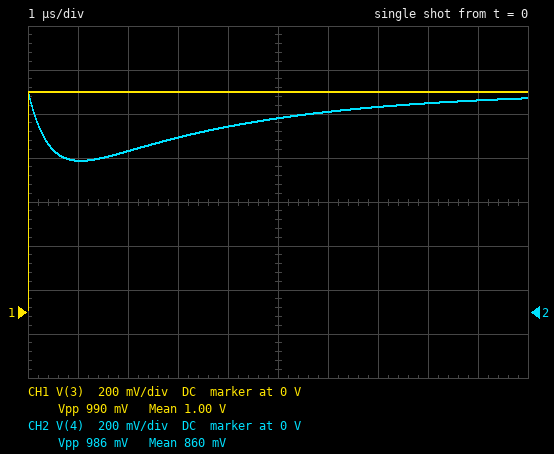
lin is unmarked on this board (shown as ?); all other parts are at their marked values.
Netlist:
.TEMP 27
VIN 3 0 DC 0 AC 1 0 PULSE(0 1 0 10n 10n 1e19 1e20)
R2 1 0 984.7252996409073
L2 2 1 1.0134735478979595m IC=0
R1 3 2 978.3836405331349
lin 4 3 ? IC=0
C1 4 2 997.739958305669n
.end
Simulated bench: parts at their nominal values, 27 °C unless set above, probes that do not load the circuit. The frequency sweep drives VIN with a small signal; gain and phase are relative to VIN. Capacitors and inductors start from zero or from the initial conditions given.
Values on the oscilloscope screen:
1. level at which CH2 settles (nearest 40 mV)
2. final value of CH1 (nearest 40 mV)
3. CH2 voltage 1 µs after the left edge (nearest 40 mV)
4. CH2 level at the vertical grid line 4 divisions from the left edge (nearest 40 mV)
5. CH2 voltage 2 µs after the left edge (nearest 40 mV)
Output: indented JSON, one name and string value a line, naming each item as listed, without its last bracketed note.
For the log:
{
  "level at which CH2 settles": "960 mV",
  "final value of CH1": "1.00 V",
  "CH2 voltage 1 µs after the left edge": "680 mV",
  "CH2 level at the vertical grid line 4 divisions from the left edge": "840 mV",
  "CH2 voltage 2 µs after the left edge": "720 mV"
}
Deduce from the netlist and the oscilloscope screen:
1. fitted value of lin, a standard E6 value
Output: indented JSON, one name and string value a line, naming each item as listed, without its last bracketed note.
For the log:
{
  "fitted value of lin, a standard E6 value": "1.5 mH"
}
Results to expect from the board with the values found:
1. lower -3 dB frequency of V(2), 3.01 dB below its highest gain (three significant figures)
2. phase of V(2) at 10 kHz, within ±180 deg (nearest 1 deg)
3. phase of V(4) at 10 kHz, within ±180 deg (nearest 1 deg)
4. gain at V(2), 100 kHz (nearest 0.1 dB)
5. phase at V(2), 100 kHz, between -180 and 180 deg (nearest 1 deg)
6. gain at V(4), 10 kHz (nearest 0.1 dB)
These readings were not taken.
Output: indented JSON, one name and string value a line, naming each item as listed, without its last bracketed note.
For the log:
{
  "lower -3 dB frequency of V(2), 3.01 dB below its highest gain": "228 Hz",
  "phase of V(2) at 10 kHz, within ±180 deg": "-4 deg",
  "phase of V(4) at 10 kHz, within ±180 deg": "-5 deg",
  "gain at V(2), 100 kHz": "-3.9 dB",
  "phase at V(2), 100 kHz, between -180 and 180 deg": "-5 deg",
  "gain at V(4), 10 kHz": "-0.1 dB"
}
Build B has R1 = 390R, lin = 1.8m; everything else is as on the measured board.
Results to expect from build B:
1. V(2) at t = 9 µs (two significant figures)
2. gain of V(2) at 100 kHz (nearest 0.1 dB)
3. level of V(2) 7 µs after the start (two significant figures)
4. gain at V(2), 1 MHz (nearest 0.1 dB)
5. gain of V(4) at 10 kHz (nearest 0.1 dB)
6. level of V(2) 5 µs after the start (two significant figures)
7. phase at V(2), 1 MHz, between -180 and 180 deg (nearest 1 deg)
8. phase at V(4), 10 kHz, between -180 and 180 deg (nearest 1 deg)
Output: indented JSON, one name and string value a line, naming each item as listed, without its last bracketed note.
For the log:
{
  "V(2) at t = 9 µs": "920 mV",
  "gain of V(2) at 100 kHz": "-2.3 dB",
  "level of V(2) 7 µs after the start": "890 mV",
  "gain at V(2), 1 MHz": "-0.1 dB",
  "gain of V(4) at 10 kHz": "-0.3 dB",
  "level of V(2) 5 µs after the start": "860 mV",
  "phase at V(2), 1 MHz, between -180 and 180 deg": "3 deg",
  "phase at V(4), 10 kHz, between -180 and 180 deg": "-6 deg"
}
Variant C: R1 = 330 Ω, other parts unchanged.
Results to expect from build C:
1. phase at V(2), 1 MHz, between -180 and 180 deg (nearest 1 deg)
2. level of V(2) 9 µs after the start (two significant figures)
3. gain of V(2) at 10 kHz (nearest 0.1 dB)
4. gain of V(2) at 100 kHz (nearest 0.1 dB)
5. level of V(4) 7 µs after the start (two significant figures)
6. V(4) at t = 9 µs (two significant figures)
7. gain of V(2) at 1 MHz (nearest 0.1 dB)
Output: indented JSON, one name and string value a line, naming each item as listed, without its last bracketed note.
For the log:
{
  "phase at V(2), 1 MHz, between -180 and 180 deg": "3 deg",
  "level of V(2) 9 µs after the start": "930 mV",
  "gain of V(2) at 10 kHz": "-0.2 dB",
  "gain of V(2) at 100 kHz": "-2.0 dB",
  "level of V(4) 7 µs after the start": "910 mV",
  "V(4) at t = 9 µs": "940 mV",
  "gain of V(2) at 1 MHz": "-0.1 dB"
}
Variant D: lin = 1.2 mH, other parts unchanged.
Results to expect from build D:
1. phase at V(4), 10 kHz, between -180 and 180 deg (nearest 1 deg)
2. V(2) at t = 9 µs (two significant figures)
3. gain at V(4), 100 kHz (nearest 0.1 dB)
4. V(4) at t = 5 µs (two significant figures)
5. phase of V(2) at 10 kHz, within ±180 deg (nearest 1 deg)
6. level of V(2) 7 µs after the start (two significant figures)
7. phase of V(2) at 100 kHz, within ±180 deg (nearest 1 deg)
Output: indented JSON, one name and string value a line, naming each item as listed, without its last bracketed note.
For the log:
{
  "phase at V(4), 10 kHz, between -180 and 180 deg": "-4 deg",
  "V(2) at t = 9 µs": "970 mV",
  "gain at V(4), 100 kHz": "-3.5 dB",
  "V(4) at t = 5 µs": "910 mV",
  "phase of V(2) at 10 kHz, within ±180 deg": "-3 deg",
  "level of V(2) 7 µs after the start": "950 mV",
  "phase of V(2) at 100 kHz, within ±180 deg": "-7 deg"
}
